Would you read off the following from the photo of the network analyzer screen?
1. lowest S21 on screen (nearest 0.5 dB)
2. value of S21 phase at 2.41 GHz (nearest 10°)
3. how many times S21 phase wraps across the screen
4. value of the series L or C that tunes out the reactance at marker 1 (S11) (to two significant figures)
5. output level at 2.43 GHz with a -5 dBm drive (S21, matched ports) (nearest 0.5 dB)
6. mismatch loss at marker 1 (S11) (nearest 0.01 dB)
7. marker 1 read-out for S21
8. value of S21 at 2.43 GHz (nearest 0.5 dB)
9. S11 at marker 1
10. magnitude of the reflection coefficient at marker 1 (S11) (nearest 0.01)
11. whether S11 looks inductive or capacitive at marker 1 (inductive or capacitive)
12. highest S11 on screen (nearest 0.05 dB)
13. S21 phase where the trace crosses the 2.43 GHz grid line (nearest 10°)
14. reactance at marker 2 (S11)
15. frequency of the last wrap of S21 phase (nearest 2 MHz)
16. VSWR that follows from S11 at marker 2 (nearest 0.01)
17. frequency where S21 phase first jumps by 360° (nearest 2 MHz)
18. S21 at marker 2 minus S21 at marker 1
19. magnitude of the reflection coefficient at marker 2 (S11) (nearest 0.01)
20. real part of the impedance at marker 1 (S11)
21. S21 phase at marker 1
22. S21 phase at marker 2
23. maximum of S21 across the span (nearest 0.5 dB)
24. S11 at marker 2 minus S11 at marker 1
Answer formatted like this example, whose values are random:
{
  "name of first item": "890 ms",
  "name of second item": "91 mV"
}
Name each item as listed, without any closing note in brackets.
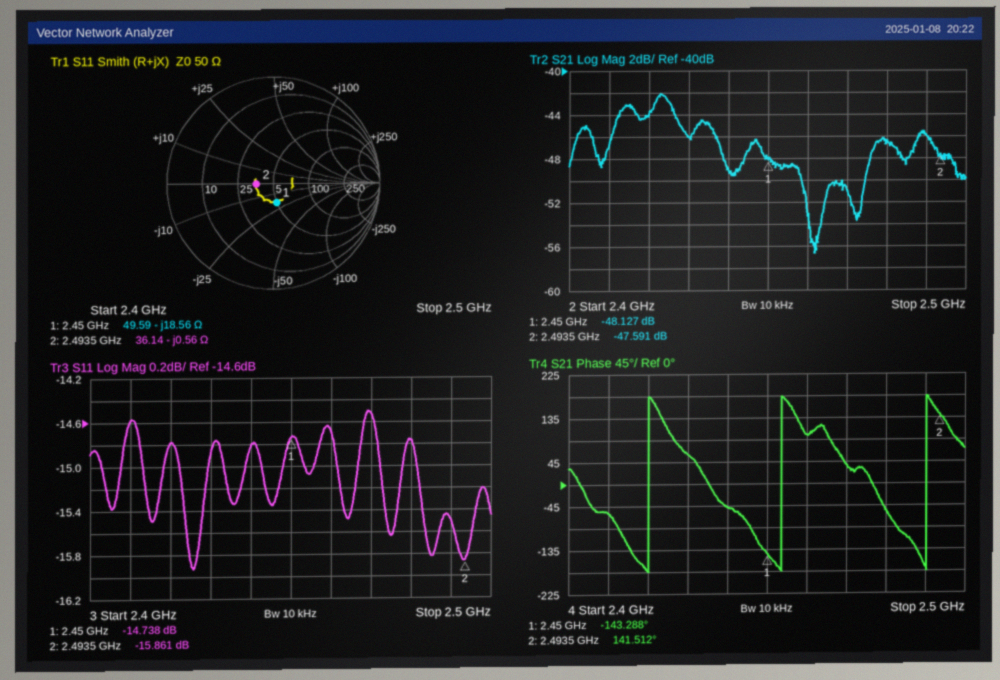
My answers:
{
  "lowest S21 on screen": "-56.5 dB",
  "value of S21 phase at 2.41 GHz": "-60°",
  "how many times S21 phase wraps across the screen": "3",
  "value of the series L or C that tunes out the reactance at marker 1 (S11)": "1.2 nH",
  "output level at 2.43 GHz with a -5 dBm drive (S21, matched ports)": "-51.0 dBm",
  "mismatch loss at marker 1 (S11)": "0.15 dB",
  "marker 1 read-out for S21": "-48.127 dB",
  "value of S21 at 2.43 GHz": "-46.0 dB",
  "S11 at marker 1": "-14.738 dB",
  "magnitude of the reflection coefficient at marker 1 (S11)": "0.18",
  "whether S11 looks inductive or capacitive at marker 1": "capacitive",
  "highest S11 on screen": "-14.50 dB",
  "S21 phase where the trace crosses the 2.43 GHz grid line": "60°",
  "reactance at marker 2": "-0.56 Ω",
  "frequency of the last wrap of S21 phase": "2.490 GHz",
  "VSWR that follows from S11 at marker 2": "1.38",
  "frequency where S21 phase first jumps by 360°": "2.420 GHz",
  "S21 at marker 2 minus S21 at marker 1": "0.536 dB",
  "magnitude of the reflection coefficient at marker 2 (S11)": "0.16",
  "real part of the impedance at marker 1": "49.59 Ω",
  "S21 phase at marker 1": "-143.288°",
  "S21 phase at marker 2": "141.512°",
  "maximum of S21 across the span": "-42.0 dB",
  "S11 at marker 2 minus S11 at marker 1": "-1.123 dB"
}
